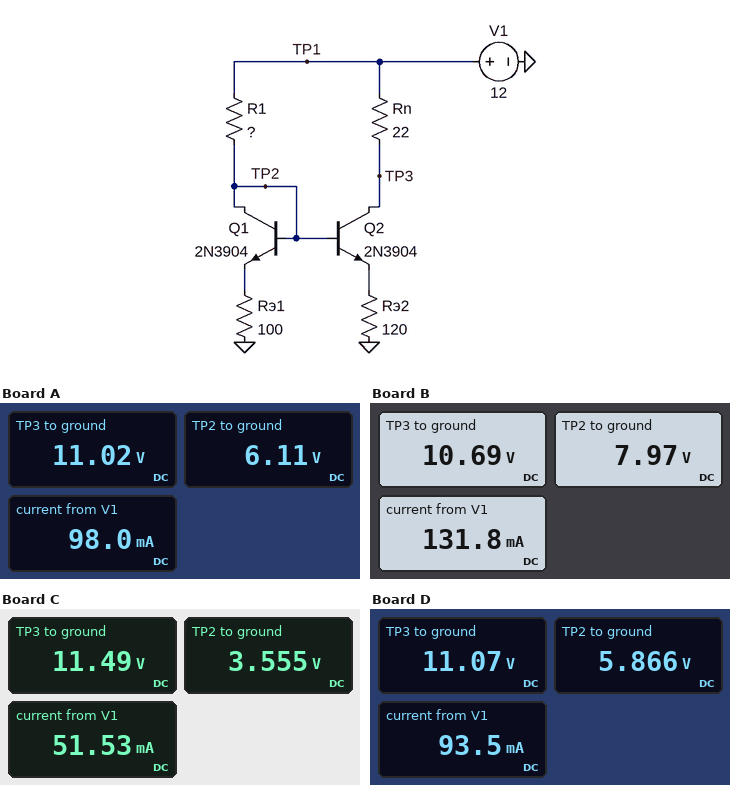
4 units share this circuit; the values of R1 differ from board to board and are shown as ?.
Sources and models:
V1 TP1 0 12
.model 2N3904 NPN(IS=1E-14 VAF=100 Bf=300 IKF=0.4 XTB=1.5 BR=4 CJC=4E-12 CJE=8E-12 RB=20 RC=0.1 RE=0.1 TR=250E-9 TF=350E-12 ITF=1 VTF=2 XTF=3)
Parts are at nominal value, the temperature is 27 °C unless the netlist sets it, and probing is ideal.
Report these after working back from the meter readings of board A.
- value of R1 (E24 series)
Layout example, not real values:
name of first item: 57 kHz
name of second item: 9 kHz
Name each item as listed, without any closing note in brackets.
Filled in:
value of R1: 110 Ω
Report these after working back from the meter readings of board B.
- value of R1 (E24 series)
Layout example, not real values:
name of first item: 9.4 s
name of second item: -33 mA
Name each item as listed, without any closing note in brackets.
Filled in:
value of R1: 56 Ω
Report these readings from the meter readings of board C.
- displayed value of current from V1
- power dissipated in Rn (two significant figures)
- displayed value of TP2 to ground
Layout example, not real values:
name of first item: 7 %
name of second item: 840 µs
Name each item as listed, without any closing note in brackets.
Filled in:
displayed value of current from V1: 51.53 mA
power dissipated in Rn: 12 mW
displayed value of TP2 to ground: 3.555 V
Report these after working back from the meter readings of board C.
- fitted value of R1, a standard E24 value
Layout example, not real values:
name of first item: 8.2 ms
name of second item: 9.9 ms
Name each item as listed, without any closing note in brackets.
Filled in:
fitted value of R1, a standard E24 value: 300 Ω
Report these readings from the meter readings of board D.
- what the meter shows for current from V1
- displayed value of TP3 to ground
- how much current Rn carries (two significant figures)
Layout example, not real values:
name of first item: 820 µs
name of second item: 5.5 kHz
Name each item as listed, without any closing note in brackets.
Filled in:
what the meter shows for current from V1: 93.5 mA
displayed value of TP3 to ground: 11.07 V
how much current Rn carries: 42 mA
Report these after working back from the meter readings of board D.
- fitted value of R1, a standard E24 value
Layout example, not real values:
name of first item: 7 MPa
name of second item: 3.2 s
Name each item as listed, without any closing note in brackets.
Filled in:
fitted value of R1, a standard E24 value: 120 Ω
